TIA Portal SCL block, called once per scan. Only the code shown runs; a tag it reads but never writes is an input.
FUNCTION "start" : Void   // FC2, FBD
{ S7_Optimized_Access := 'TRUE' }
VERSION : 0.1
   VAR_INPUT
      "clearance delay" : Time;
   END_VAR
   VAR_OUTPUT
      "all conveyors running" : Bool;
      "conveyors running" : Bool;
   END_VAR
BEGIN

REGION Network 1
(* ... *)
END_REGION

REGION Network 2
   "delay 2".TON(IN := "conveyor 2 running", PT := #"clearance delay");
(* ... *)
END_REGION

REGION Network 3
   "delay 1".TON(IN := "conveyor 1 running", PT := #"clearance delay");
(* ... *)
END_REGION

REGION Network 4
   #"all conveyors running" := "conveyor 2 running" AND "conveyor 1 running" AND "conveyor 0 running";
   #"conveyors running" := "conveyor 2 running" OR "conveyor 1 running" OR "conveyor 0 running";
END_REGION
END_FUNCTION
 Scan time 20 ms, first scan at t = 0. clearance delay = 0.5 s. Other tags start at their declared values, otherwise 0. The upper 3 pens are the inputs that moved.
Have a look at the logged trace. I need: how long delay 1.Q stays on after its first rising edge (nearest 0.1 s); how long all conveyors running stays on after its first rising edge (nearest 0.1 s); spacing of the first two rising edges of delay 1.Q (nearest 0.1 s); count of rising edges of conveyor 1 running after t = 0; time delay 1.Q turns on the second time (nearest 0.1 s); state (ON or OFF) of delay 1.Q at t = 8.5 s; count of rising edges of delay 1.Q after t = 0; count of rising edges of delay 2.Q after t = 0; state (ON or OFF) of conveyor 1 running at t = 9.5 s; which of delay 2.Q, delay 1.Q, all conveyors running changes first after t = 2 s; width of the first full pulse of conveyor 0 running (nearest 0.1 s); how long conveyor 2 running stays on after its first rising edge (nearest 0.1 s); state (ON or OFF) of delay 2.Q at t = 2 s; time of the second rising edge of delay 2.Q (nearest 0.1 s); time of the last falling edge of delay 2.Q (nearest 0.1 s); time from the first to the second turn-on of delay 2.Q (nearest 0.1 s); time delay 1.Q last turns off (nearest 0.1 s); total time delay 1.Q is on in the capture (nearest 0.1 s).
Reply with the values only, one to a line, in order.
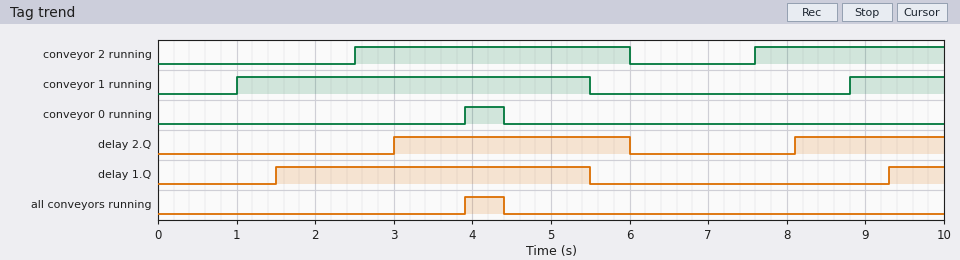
4.0 s
0.5 s
7.8 s
2
9.3 s
OFF
2
2
ON
delay 2.Q
0.5 s
3.5 s
OFF
8.1 s
6.0 s
5.1 s
5.5 s
4.7 s
